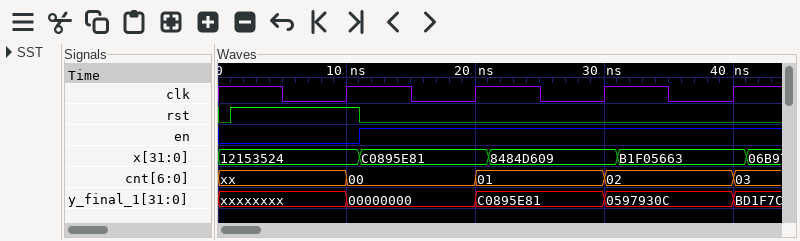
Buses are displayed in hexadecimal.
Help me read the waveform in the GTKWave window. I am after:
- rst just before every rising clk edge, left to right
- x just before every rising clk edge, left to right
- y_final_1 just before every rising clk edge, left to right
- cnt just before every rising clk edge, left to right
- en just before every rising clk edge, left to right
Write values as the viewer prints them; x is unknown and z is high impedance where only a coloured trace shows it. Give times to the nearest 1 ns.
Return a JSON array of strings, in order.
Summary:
["1 0 0 0", "12153524, C0895E81, 8484D609, B1F05663", "xxxxxxxx, 00000000, C0895E81, 0597930C", "xx, 00, 01, 02", "0 1 1 1"]
